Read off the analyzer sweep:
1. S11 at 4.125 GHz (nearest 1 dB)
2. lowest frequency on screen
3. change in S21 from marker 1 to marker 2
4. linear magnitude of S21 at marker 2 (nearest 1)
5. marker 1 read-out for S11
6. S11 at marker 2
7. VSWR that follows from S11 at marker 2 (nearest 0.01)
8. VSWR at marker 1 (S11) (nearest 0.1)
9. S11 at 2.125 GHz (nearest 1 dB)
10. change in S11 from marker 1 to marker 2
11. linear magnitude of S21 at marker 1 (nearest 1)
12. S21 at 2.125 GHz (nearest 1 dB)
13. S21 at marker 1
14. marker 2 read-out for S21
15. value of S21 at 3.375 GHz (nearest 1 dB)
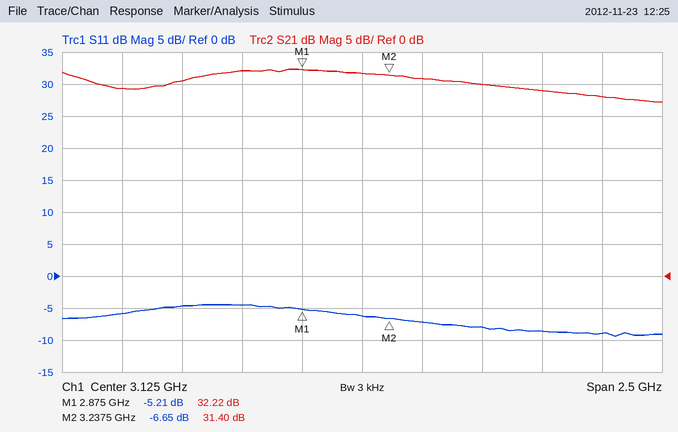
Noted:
-9 dB
1.875 GHz
-0.82 dB
37
-5.21 dB
-6.65 dB
2.74
3.4
-6 dB
-1.44 dB
41
29 dB
32.22 dB
31.40 dB
31 dB
